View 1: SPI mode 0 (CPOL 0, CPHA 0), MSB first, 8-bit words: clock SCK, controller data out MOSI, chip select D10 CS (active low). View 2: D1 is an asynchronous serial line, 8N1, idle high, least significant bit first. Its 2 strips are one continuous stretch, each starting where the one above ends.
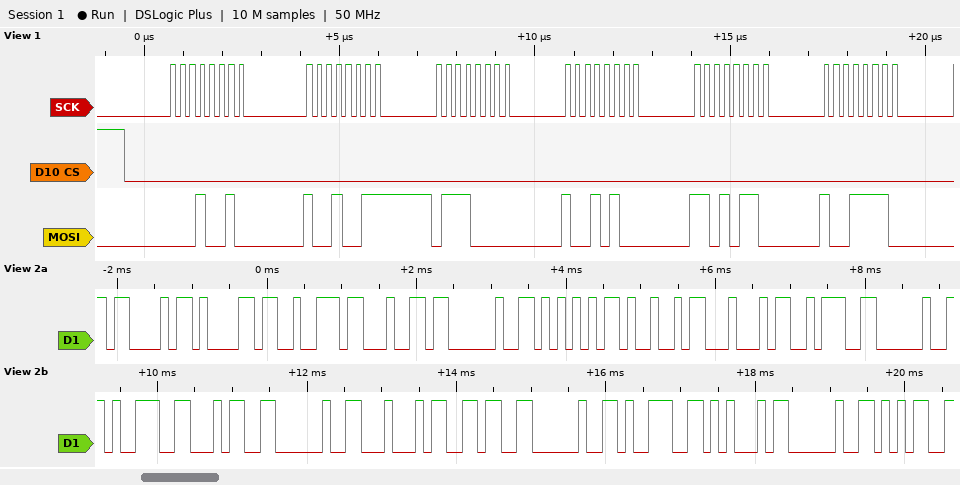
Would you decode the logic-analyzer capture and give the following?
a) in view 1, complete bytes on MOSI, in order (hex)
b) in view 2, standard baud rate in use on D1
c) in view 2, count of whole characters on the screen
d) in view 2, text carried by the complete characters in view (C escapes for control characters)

12 93 70 94 D6 9E
9600 baud
20
"Card UID: 94 D6 9E 5"
